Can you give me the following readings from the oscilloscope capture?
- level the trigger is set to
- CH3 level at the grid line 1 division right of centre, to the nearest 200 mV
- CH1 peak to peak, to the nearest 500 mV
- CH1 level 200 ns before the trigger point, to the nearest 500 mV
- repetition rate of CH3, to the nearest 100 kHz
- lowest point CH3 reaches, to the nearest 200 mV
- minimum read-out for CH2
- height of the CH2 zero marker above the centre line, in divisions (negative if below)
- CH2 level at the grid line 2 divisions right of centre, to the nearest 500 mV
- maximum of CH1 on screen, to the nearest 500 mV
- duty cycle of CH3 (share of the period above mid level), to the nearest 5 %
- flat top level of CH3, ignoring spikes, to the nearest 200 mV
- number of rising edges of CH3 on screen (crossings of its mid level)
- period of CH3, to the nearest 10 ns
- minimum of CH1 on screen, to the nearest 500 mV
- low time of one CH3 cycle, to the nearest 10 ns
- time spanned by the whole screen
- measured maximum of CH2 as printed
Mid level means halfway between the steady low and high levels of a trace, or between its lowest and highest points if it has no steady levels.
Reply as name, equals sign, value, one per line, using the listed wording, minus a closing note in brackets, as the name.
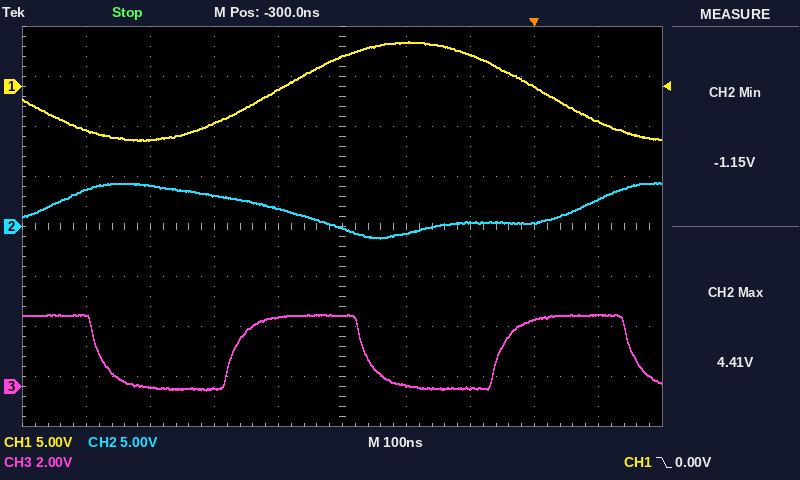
level the trigger is set to = 0.00 V
CH3 level at the grid line 1 division right of centre, to the nearest 200 mV = 0.0 V
CH1 peak to peak, to the nearest 500 mV = 10.0 V
CH1 level 200 ns before the trigger point, to the nearest 500 mV = 4.5 V
repetition rate of CH3, to the nearest 100 kHz = 2.4 MHz
lowest point CH3 reaches, to the nearest 200 mV = -200 mV
minimum read-out for CH2 = -1.15 V
height of the CH2 zero marker above the centre line, in divisions = 0.0 div
CH2 level at the grid line 2 divisions right of centre, to the nearest 500 mV = 500 mV
maximum of CH1 on screen, to the nearest 500 mV = 4.5 V
duty cycle of CH3 (share of the period above mid level), to the nearest 5 % = 50 %
flat top level of CH3, ignoring spikes, to the nearest 200 mV = 2.8 V
number of rising edges of CH3 on screen = 2
period of CH3, to the nearest 10 ns = 420 ns
minimum of CH1 on screen, to the nearest 500 mV = -5.5 V
low time of one CH3 cycle, to the nearest 10 ns = 210 ns
time spanned by the whole screen = 1 µs
measured maximum of CH2 as printed = 4.41 V
